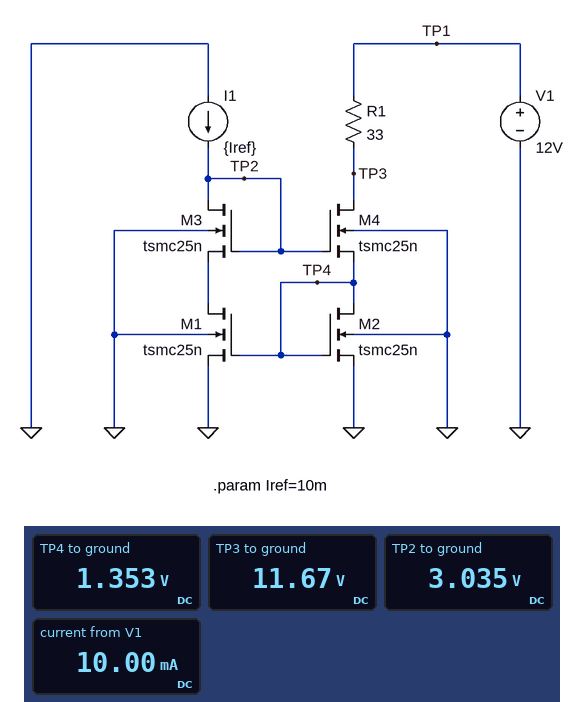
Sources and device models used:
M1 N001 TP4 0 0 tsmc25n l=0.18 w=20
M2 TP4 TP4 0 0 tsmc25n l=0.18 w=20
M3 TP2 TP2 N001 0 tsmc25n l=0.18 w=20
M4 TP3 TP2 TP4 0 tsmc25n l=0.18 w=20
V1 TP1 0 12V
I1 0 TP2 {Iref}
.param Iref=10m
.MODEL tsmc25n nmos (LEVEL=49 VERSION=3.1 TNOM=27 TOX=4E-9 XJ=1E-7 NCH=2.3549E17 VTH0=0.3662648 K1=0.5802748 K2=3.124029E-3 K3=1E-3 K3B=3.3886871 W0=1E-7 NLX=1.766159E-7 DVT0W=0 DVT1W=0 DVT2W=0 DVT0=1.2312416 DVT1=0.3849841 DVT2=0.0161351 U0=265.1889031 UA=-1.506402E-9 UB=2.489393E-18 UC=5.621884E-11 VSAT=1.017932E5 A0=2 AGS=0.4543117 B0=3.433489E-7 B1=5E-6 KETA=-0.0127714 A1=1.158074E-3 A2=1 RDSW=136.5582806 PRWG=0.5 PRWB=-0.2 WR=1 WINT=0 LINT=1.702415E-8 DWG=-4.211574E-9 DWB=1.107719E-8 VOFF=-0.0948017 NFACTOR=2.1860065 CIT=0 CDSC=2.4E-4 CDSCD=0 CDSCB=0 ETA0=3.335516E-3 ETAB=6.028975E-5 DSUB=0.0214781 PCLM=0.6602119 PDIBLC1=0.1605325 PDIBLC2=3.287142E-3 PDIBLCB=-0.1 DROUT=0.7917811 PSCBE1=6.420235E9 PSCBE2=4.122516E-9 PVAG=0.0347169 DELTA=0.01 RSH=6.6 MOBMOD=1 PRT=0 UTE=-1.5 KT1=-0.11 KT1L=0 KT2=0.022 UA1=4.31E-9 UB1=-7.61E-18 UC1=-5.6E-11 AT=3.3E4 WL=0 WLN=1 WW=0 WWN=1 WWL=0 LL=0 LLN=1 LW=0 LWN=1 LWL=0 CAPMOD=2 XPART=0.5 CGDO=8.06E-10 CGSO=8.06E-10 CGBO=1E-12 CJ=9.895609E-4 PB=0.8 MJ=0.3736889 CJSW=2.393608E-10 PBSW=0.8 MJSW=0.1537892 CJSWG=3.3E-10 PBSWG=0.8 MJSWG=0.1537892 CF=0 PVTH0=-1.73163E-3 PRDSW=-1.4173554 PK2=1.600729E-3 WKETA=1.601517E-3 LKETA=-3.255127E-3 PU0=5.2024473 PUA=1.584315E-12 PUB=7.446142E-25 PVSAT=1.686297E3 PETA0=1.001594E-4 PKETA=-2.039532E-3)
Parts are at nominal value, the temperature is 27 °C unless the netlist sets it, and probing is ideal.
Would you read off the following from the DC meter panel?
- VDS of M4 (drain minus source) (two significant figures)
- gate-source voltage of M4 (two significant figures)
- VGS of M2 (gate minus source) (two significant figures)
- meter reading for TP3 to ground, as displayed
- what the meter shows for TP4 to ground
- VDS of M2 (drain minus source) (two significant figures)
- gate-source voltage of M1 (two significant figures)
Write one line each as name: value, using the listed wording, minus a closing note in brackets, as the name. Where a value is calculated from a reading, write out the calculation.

VDS of M4 (drain minus source): 11.67 V - 1.353 V = 10 V
gate-source voltage of M4: 3.035 V - 1.353 V = 1.7 V
VGS of M2 (gate minus source): 1.353 V = 1.4 V
meter reading for TP3 to ground, as displayed: 11.67 V
what the meter shows for TP4 to ground: 1.353 V
VDS of M2 (drain minus source): 1.353 V = 1.4 V
gate-source voltage of M1: 1.353 V = 1.4 V
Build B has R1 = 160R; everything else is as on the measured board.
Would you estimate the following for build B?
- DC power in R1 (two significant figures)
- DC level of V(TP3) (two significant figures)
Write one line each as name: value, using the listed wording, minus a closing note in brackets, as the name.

DC power in R1: 16 mW
DC level of V(TP3): 10 V
